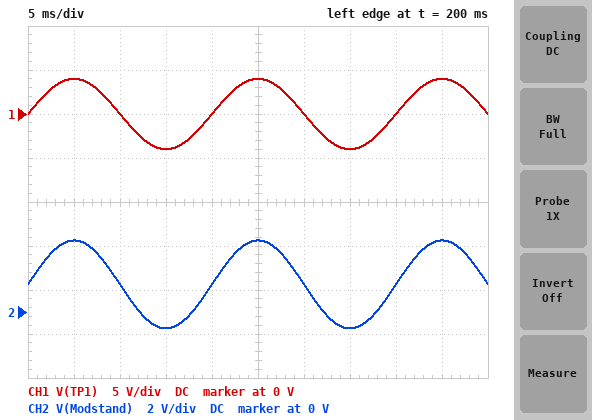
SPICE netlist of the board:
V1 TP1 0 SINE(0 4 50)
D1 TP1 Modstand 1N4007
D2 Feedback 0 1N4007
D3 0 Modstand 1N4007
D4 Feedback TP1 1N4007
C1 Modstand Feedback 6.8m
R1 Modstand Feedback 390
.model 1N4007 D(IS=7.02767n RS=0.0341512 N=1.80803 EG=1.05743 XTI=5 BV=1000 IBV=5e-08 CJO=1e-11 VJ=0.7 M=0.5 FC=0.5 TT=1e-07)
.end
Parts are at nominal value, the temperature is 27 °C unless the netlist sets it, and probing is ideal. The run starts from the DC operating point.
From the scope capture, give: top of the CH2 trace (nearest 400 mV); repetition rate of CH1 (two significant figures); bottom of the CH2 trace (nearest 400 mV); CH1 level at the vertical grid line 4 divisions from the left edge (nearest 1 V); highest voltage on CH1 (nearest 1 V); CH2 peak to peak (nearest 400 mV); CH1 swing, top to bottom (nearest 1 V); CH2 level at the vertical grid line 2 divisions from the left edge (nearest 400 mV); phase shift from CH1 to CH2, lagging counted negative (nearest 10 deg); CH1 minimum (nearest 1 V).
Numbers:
3.2 V
50 Hz
-800 mV
0 V
4 V
4.0 V
8 V
1.2 V
0 deg
-4 V
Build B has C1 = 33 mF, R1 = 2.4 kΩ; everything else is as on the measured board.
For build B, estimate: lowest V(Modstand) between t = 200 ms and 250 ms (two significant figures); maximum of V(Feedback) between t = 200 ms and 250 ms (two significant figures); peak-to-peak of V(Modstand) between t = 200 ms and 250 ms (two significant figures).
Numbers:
-800 mV
800 mV
4.0 V
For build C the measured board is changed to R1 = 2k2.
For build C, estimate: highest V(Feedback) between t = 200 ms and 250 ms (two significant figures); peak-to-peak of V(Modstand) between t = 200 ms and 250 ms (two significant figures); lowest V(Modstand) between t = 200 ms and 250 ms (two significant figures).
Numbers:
720 mV
4.0 V
-720 mV
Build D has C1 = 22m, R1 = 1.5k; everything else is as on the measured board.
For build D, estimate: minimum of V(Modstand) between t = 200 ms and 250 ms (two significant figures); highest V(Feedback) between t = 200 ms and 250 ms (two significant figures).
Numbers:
-770 mV
780 mV
